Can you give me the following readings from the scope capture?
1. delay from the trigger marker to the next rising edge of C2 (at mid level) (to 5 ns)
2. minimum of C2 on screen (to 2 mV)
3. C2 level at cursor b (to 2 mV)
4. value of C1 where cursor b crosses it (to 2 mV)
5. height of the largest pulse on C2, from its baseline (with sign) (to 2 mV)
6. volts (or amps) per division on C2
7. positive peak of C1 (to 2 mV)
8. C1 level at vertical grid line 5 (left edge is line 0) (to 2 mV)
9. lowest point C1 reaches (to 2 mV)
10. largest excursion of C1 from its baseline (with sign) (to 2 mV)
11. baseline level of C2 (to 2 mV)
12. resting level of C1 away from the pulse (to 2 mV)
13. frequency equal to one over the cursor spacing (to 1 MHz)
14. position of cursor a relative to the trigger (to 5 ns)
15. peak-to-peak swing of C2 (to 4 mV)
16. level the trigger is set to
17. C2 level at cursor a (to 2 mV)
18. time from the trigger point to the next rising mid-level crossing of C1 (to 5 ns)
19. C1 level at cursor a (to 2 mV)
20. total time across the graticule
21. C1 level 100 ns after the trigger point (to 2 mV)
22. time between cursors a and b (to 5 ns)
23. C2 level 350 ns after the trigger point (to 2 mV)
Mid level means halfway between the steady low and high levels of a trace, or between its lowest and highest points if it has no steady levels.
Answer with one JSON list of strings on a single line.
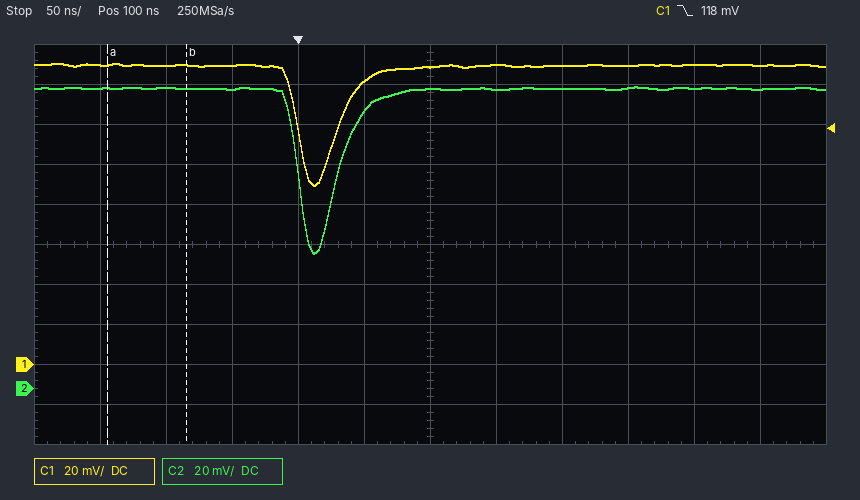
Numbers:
["30 ns", "68 mV", "150 mV", "150 mV", "-82 mV", "20 mV", "150 mV", "142 mV", "90 mV", "-60 mV", "150 mV", "150 mV", "17 MHz", "-145 ns", "84 mV", "118 mV", "150 mV", "30 ns", "150 mV", "600 ns", "148 mV", "60 ns", "150 mV"]
